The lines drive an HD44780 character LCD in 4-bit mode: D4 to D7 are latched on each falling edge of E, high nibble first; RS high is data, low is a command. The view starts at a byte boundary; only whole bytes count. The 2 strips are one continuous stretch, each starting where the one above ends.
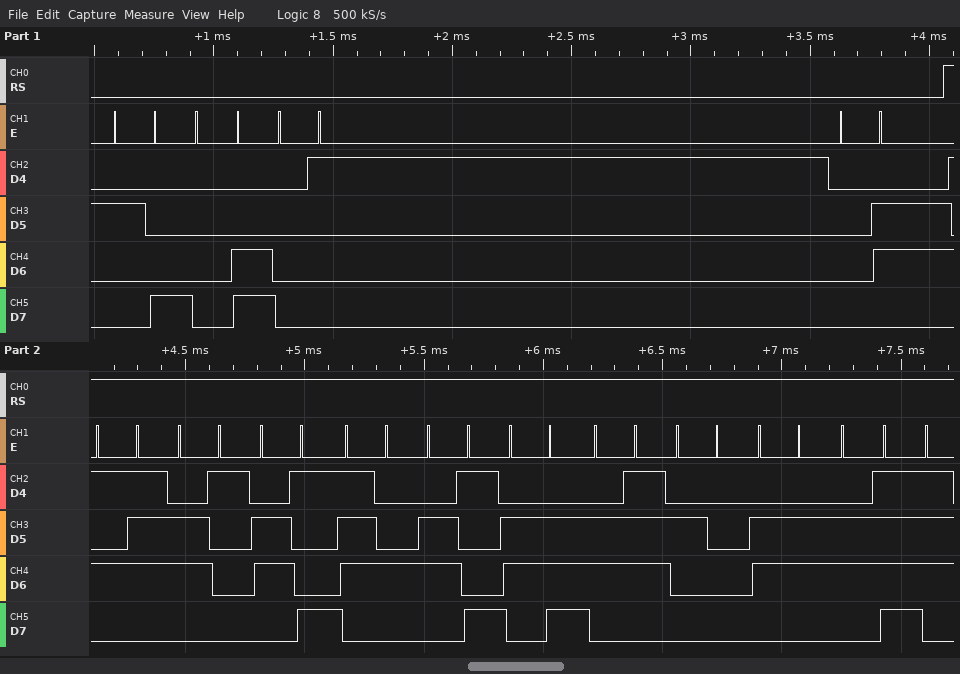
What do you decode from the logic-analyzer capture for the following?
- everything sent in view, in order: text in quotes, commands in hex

0x28 0x0C 0x01 0x06 "Waiting fo"
